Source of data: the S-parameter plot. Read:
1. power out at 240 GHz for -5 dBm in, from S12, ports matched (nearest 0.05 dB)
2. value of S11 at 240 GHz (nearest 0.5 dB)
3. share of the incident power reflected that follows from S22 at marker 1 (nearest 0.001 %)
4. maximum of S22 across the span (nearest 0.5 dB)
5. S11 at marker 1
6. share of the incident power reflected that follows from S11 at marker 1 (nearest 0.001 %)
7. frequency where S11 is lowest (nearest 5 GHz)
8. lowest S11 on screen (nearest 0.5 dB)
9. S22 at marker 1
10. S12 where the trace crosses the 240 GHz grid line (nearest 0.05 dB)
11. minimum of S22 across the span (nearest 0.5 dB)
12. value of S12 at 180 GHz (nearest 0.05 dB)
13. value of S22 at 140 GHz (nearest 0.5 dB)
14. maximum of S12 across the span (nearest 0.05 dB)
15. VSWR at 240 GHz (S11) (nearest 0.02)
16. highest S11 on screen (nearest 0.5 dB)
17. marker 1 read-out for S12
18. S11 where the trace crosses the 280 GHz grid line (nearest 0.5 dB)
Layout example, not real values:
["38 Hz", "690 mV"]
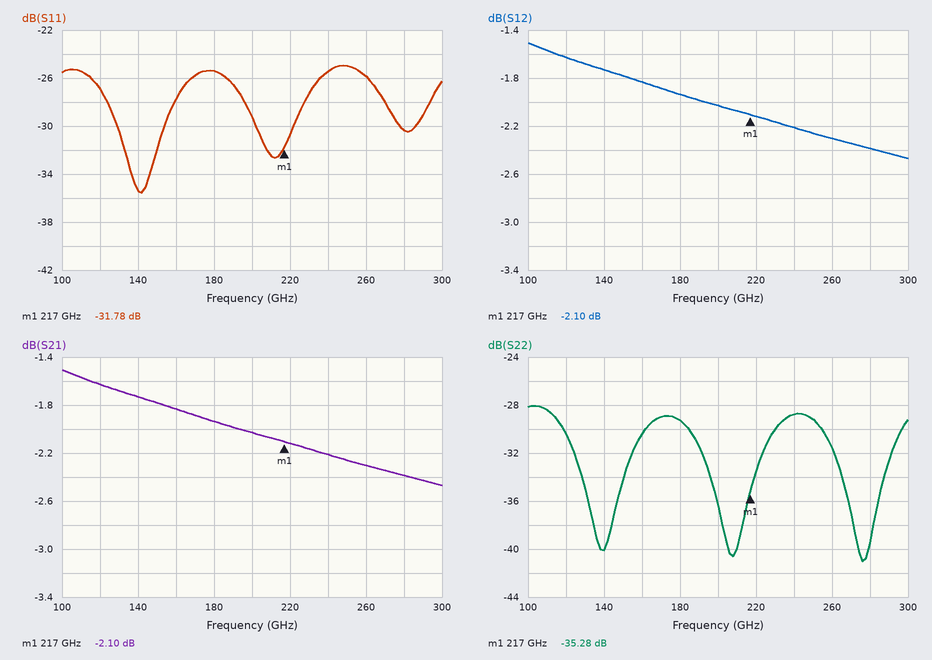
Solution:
["-7.20 dBm", "-25.5 dB", "0.030 %", "-28.0 dB", "-31.78 dB", "0.066 %", "140 GHz", "-35.5 dB", "-35.28 dB", "-2.20 dB", "-41.0 dB", "-1.95 dB", "-40.0 dB", "-1.50 dB", "1.12", "-25.0 dB", "-2.10 dB", "-30.5 dB"]
